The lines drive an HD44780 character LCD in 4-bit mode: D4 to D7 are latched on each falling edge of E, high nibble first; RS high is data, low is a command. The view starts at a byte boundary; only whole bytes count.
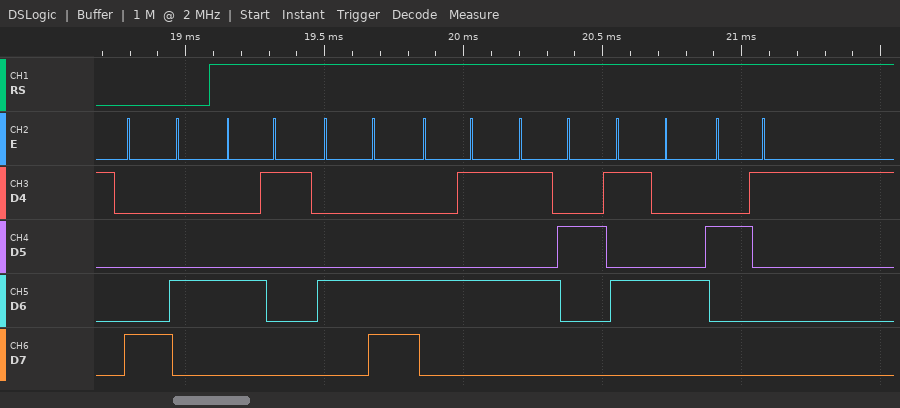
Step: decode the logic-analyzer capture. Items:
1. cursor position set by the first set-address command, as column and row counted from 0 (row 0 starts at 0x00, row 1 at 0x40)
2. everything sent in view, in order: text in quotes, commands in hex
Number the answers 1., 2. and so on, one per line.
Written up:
1. column 4, row 0
2. 0x84 "ALERT!"
